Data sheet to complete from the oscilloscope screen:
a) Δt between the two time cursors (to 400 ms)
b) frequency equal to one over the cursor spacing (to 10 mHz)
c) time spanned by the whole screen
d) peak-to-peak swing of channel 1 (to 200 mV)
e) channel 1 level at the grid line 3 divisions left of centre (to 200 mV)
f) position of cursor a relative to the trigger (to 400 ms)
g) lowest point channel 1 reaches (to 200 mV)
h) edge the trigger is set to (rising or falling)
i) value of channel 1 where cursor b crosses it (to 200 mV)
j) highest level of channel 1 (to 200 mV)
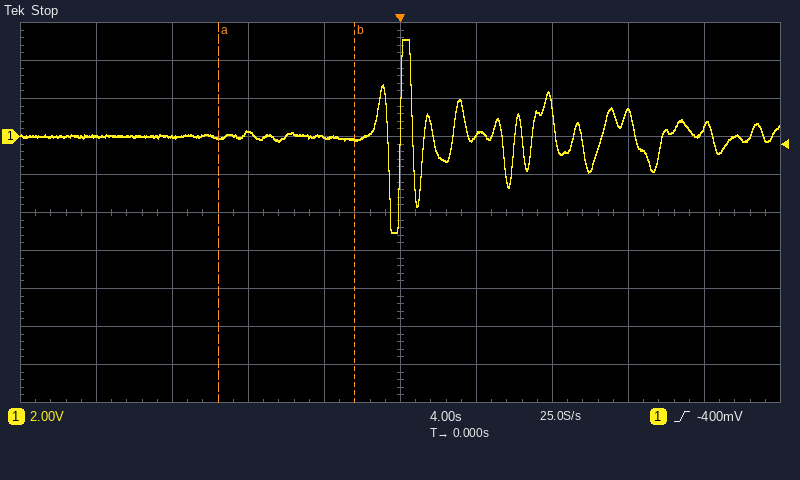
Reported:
7.2 s
140 mHz
40 s
10.2 V
0.0 V
-9.6 s
-5.0 V
rising
-200 mV
5.2 V
